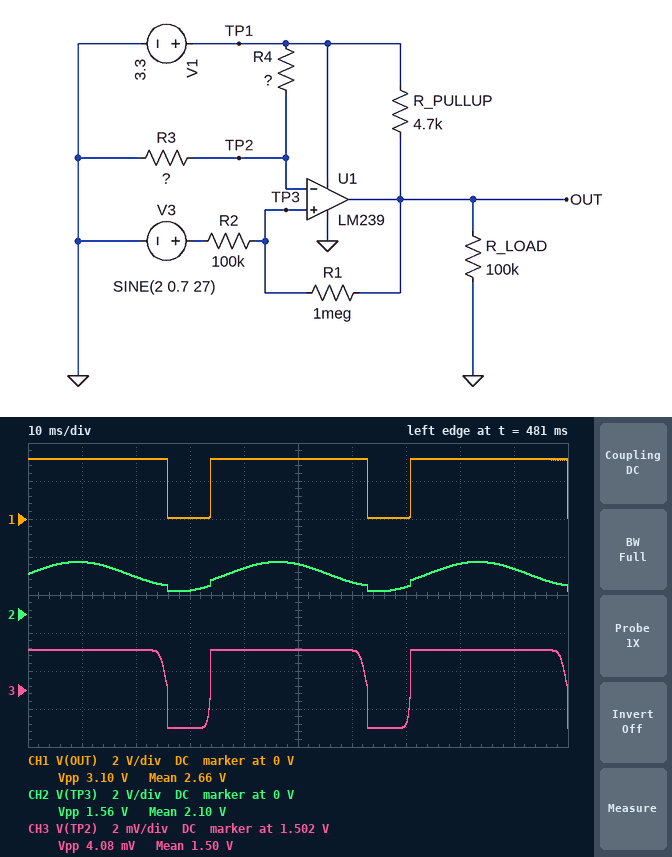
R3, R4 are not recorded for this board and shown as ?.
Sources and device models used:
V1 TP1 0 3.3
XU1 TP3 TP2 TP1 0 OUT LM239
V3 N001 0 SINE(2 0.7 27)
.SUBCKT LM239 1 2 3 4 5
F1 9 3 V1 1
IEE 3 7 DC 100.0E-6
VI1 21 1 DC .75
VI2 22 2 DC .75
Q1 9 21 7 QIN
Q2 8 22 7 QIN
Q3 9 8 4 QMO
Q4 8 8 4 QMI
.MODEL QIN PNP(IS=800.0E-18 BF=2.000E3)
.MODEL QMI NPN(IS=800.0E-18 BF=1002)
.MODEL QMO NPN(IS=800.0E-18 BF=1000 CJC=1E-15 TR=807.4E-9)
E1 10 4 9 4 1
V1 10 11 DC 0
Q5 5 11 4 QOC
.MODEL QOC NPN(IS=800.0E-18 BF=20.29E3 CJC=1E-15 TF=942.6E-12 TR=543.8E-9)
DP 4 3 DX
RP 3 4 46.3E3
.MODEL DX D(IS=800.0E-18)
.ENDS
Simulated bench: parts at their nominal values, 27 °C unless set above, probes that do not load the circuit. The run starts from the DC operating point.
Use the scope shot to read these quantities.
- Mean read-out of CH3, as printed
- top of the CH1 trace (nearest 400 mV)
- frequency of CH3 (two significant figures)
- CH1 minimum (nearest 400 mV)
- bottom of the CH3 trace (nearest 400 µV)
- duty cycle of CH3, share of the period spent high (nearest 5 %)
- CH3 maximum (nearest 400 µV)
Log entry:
1.50 V
3.2 V
27 Hz
0 V
1.5000 V
80 %
1.5040 V
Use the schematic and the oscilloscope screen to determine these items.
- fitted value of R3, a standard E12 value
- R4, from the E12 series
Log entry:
150 kΩ
180 kΩ
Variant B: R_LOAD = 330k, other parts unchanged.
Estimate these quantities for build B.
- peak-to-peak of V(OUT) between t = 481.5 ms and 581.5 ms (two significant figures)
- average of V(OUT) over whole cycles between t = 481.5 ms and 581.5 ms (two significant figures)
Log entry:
3.2 V
2.6 V
